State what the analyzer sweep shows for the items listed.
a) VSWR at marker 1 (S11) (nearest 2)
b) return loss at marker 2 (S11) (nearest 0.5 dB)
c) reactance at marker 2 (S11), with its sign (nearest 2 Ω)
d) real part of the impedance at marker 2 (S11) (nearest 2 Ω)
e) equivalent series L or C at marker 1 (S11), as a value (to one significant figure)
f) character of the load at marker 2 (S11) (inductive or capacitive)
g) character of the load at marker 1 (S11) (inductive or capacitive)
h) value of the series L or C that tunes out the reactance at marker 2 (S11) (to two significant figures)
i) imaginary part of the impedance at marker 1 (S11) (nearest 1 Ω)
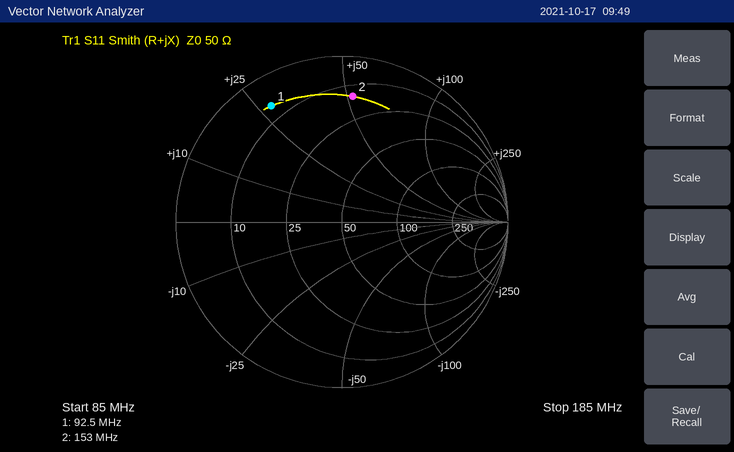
10
2.5 dB
+52 Ω
14 Ω
50 nH
inductive
inductive
20 pF
+28 Ω
